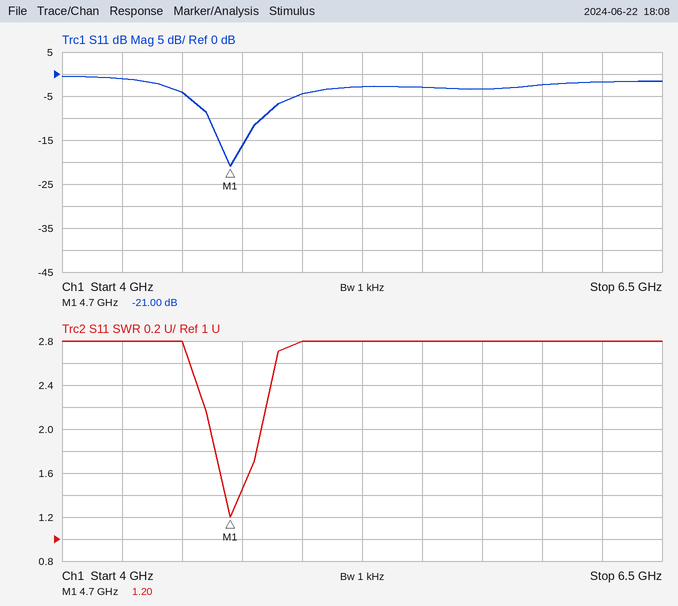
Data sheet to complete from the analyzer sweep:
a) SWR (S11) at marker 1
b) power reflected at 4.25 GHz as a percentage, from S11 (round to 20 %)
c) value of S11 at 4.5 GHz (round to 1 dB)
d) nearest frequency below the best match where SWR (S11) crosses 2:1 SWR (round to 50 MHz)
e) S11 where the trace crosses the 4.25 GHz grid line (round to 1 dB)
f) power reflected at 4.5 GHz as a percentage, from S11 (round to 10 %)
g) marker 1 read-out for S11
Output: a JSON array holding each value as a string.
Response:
["1.20", "80 %", "-4 dB", "4.60 GHz", "-1 dB", "40 %", "-21.00 dB"]
